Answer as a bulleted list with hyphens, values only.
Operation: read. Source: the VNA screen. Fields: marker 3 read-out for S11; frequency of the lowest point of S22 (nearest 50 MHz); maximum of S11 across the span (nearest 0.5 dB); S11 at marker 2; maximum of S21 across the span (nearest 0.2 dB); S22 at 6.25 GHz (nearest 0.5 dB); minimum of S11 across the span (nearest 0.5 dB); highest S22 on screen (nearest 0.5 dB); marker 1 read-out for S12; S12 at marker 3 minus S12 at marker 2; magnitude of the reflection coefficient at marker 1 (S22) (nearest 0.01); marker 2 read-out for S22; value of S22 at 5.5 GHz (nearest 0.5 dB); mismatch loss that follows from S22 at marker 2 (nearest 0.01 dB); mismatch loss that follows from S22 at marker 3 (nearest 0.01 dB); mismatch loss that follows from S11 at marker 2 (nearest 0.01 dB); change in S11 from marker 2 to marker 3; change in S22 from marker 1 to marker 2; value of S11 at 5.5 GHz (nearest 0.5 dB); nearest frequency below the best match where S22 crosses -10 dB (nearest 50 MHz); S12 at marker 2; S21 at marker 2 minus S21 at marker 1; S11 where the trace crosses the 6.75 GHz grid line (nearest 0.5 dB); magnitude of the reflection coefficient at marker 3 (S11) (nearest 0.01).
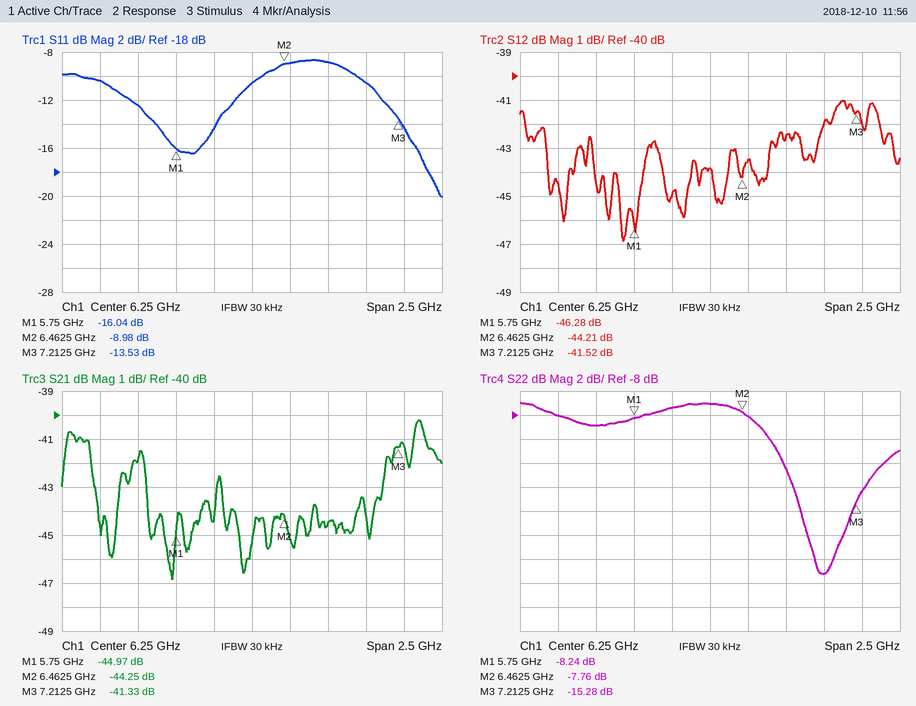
- -13.53 dB
- 7.00 GHz
- -8.5 dB
- -8.98 dB
- -40.2 dB
- -7.0 dB
- -20.0 dB
- -7.0 dB
- -46.28 dB
- 2.69 dB
- 0.39
- -7.76 dB
- -9.0 dB
- 0.80 dB
- 0.13 dB
- 0.59 dB
- -4.55 dB
- 0.48 dB
- -12.5 dB
- 6.65 GHz
- -44.21 dB
- 0.72 dB
- -9.0 dB
- 0.21
